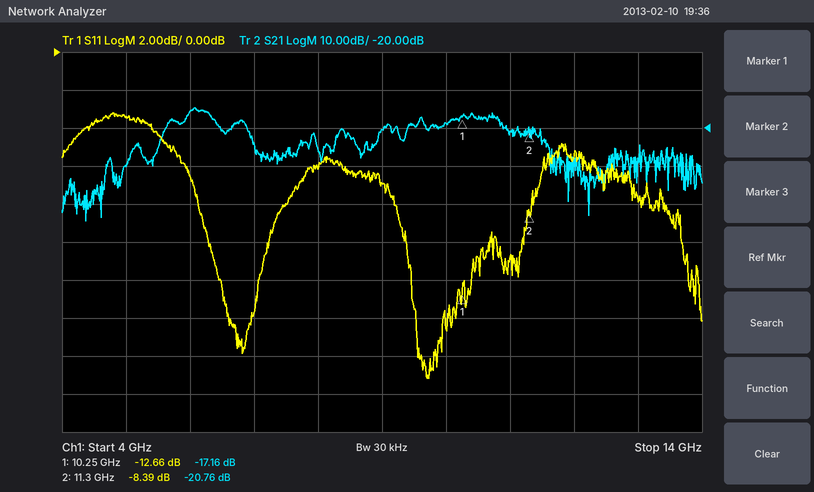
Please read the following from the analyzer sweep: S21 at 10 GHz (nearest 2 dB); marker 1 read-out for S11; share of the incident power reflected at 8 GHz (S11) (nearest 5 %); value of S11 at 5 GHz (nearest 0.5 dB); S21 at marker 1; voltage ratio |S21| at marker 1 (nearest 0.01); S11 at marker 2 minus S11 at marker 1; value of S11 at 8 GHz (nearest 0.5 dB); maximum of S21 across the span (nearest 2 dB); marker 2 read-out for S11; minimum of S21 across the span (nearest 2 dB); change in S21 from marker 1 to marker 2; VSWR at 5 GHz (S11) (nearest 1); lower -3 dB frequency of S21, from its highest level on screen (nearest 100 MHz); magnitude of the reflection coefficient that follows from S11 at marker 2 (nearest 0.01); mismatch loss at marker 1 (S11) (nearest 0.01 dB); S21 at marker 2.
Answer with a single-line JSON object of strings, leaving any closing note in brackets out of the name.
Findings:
{"S21 at 10 GHz": "-18 dB", "marker 1 read-out for S11": "-12.66 dB", "share of the incident power reflected at 8 GHz (S11)": "25 %", "value of S11 at 5 GHz": "-3.5 dB", "S21 at marker 1": "-17.16 dB", "voltage ratio |S21| at marker 1": "0.14", "S11 at marker 2 minus S11 at marker 1": "4.27 dB", "value of S11 at 8 GHz": "-6.0 dB", "maximum of S21 across the span": "-14 dB", "marker 2 read-out for S11": "-8.39 dB", "minimum of S21 across the span": "-44 dB", "change in S21 from marker 1 to marker 2": "-3.60 dB", "VSWR at 5 GHz (S11)": "5", "lower -3 dB frequency of S21, from its highest level on screen": "5.9 GHz", "magnitude of the reflection coefficient that follows from S11 at marker 2": "0.38", "mismatch loss at marker 1 (S11)": "0.24 dB", "S21 at marker 2": "-20.76 dB"}
